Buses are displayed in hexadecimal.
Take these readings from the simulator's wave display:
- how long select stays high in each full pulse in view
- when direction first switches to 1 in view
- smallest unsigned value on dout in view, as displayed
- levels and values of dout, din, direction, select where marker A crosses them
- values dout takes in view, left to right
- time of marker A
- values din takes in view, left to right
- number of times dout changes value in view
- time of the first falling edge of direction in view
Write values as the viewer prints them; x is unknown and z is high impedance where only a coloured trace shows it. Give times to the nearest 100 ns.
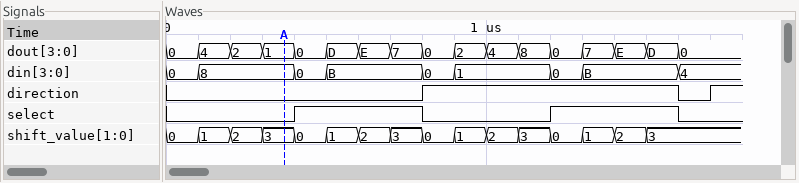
400 ns, 400 ns
800 ns
0
dout=1, din=8, direction=0, select=0
0, 4, 2, 1, 0, D, E, 7, 0, 2, 4, 8, 0, 7, E, D, 0
400 ns
0, 8, 0, B, 0, 1, 0, B, 4
16
1600 ns
